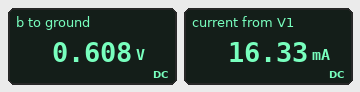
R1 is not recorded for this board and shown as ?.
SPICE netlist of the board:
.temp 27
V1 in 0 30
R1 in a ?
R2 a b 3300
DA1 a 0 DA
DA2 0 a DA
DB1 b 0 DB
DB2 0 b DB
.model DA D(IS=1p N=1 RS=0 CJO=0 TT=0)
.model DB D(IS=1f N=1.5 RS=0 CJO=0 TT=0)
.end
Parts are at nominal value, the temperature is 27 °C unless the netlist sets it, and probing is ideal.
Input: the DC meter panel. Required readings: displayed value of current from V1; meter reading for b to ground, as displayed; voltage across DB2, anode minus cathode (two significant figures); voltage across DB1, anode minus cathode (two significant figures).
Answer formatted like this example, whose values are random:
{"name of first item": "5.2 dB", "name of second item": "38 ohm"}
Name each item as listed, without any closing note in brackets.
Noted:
{"displayed value of current from V1": "16.33 mA", "meter reading for b to ground, as displayed": "0.608 V", "voltage across DB2, anode minus cathode": "-610 mV", "voltage across DB1, anode minus cathode": "610 mV"}
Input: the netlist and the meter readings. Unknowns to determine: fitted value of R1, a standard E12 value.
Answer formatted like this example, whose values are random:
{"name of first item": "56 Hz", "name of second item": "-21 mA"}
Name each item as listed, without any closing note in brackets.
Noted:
{"fitted value of R1, a standard E12 value": "1.8 kΩ"}
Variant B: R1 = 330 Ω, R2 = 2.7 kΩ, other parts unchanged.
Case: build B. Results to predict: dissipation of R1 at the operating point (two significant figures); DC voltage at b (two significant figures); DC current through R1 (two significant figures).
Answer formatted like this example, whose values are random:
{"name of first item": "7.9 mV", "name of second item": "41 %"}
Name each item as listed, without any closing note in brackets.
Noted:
{"dissipation of R1 at the operating point": "2.6 W", "DC voltage at b": "650 mV", "DC current through R1": "89 mA"}
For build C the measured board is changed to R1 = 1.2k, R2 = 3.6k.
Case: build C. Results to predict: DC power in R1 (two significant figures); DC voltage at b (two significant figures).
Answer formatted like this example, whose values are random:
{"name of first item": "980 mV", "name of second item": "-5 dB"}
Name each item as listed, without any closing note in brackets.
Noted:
{"DC power in R1": "720 mW", "DC voltage at b": "620 mV"}
